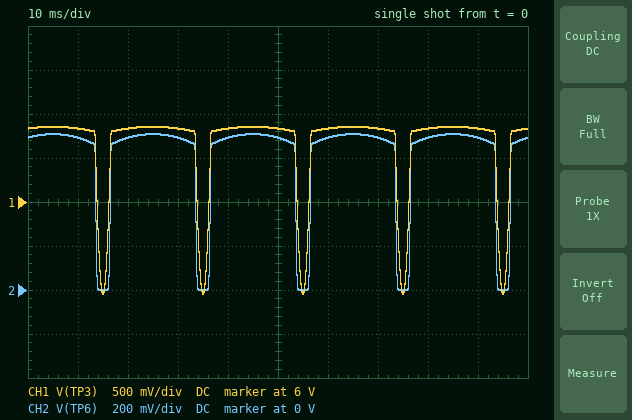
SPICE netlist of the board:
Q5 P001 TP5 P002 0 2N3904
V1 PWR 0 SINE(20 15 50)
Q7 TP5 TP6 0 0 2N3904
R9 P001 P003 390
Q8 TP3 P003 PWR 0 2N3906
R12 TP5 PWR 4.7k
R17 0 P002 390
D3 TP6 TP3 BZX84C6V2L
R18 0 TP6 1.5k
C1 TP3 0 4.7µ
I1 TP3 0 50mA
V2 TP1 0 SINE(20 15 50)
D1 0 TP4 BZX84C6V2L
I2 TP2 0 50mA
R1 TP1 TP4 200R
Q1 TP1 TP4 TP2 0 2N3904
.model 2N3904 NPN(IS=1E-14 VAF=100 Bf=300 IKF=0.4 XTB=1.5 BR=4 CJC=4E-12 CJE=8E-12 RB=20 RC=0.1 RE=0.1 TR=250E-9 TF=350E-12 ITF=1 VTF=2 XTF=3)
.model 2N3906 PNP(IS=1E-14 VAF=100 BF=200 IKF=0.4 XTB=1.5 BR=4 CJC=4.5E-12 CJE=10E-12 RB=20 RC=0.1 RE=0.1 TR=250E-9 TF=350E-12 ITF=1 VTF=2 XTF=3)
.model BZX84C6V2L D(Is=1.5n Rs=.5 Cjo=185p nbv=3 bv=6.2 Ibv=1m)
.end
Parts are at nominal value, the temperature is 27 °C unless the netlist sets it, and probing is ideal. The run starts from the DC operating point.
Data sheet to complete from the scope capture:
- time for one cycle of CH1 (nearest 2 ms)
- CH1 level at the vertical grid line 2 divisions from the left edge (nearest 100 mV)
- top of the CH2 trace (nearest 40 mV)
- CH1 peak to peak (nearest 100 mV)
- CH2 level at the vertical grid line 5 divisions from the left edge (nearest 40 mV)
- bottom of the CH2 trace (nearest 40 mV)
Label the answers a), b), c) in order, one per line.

a) 20 ms
b) 6.8 V
c) 720 mV
d) 1.9 V
e) 680 mV
f) 0 V
